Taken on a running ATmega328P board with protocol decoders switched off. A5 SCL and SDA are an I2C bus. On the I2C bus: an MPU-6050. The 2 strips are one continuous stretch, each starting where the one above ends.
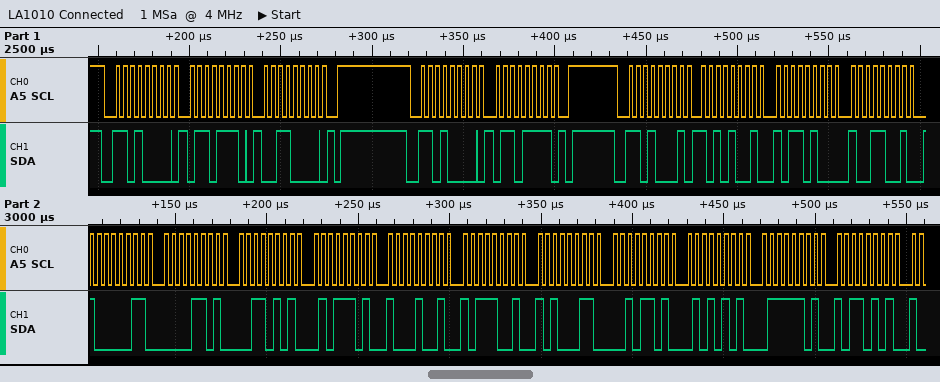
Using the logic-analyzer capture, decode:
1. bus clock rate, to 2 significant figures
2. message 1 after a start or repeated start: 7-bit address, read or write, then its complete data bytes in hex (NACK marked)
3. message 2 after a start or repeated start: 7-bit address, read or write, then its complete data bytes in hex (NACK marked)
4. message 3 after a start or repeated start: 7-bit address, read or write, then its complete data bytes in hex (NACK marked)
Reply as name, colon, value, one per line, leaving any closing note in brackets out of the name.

bus clock rate, to 2 significant figures: 250 kHz
message 1 after a start or repeated start: 7-bit address, read or write, then its complete data bytes in hex: 0x68 write: 6E 30
message 2 after a start or repeated start: 7-bit address, read or write, then its complete data bytes in hex: 0x68 write: 6F
message 3 after a start or repeated start: 7-bit address, read or write, then its complete data bytes in hex: 0x68 read: A9 B4 99 83 0D 35 5D 89 B9 A3 2D 55 7D B5
